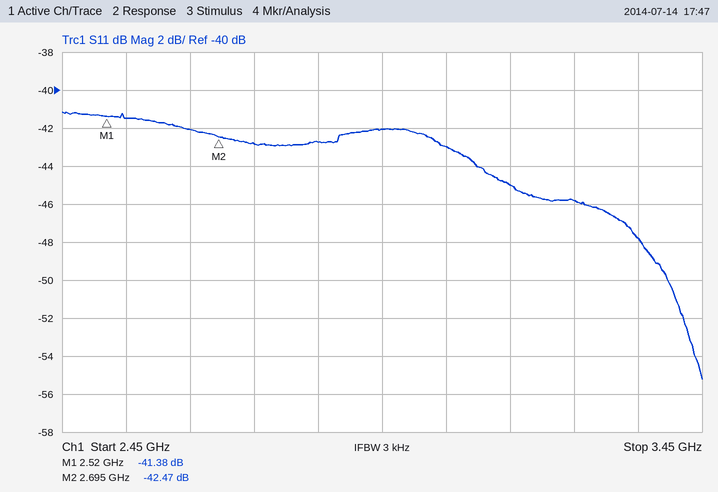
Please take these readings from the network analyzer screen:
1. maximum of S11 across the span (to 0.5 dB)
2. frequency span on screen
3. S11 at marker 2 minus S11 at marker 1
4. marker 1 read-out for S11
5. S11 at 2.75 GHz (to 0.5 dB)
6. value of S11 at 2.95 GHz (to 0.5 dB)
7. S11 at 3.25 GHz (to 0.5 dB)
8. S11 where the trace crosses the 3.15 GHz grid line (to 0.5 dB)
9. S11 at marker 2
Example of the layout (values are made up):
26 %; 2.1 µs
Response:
-41.0 dB; 1 GHz; -1.09 dB; -41.38 dB; -43.0 dB; -42.0 dB; -46.0 dB; -45.0 dB; -42.47 dB
